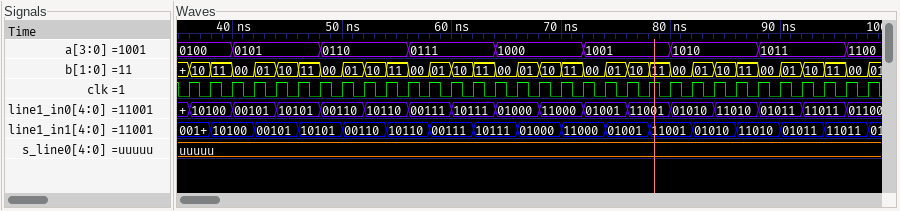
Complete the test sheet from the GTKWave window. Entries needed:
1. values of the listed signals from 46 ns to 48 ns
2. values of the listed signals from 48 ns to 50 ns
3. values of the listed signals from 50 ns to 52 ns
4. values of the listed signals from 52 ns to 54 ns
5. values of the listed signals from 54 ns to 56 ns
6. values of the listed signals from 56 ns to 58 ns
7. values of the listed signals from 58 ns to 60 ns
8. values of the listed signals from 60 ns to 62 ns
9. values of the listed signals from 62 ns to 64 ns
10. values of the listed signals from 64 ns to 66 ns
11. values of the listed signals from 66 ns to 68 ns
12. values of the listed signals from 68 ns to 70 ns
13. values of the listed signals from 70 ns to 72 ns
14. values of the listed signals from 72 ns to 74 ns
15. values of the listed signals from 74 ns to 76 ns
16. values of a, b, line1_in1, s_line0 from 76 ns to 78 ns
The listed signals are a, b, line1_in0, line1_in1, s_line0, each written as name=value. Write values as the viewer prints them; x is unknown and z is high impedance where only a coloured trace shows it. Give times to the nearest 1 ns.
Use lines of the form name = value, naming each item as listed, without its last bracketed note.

values of the listed signals from 46 ns to 48 ns = a=0101, b=11, line1_in0=10101, line1_in1=10101, s_line0=uuuuu
values of the listed signals from 48 ns to 50 ns = a=0110, b=00, line1_in0=00110, line1_in1=10101, s_line0=uuuuu
values of the listed signals from 50 ns to 52 ns = a=0110, b=01, line1_in0=00110, line1_in1=00110, s_line0=uuuuu
values of the listed signals from 52 ns to 54 ns = a=0110, b=10, line1_in0=10110, line1_in1=00110, s_line0=uuuuu
values of the listed signals from 54 ns to 56 ns = a=0110, b=11, line1_in0=10110, line1_in1=10110, s_line0=uuuuu
values of the listed signals from 56 ns to 58 ns = a=0111, b=00, line1_in0=00111, line1_in1=10110, s_line0=uuuuu
values of the listed signals from 58 ns to 60 ns = a=0111, b=01, line1_in0=00111, line1_in1=00111, s_line0=uuuuu
values of the listed signals from 60 ns to 62 ns = a=0111, b=10, line1_in0=10111, line1_in1=00111, s_line0=uuuuu
values of the listed signals from 62 ns to 64 ns = a=0111, b=11, line1_in0=10111, line1_in1=10111, s_line0=uuuuu
values of the listed signals from 64 ns to 66 ns = a=1000, b=00, line1_in0=01000, line1_in1=10111, s_line0=uuuuu
values of the listed signals from 66 ns to 68 ns = a=1000, b=01, line1_in0=01000, line1_in1=01000, s_line0=uuuuu
values of the listed signals from 68 ns to 70 ns = a=1000, b=10, line1_in0=11000, line1_in1=01000, s_line0=uuuuu
values of the listed signals from 70 ns to 72 ns = a=1000, b=11, line1_in0=11000, line1_in1=11000, s_line0=uuuuu
values of the listed signals from 72 ns to 74 ns = a=1001, b=00, line1_in0=01001, line1_in1=11000, s_line0=uuuuu
values of the listed signals from 74 ns to 76 ns = a=1001, b=01, line1_in0=01001, line1_in1=01001, s_line0=uuuuu
values of a, b, line1_in1, s_line0 from 76 ns to 78 ns = a=1001, b=10, line1_in1=01001, s_line0=uuuuu
